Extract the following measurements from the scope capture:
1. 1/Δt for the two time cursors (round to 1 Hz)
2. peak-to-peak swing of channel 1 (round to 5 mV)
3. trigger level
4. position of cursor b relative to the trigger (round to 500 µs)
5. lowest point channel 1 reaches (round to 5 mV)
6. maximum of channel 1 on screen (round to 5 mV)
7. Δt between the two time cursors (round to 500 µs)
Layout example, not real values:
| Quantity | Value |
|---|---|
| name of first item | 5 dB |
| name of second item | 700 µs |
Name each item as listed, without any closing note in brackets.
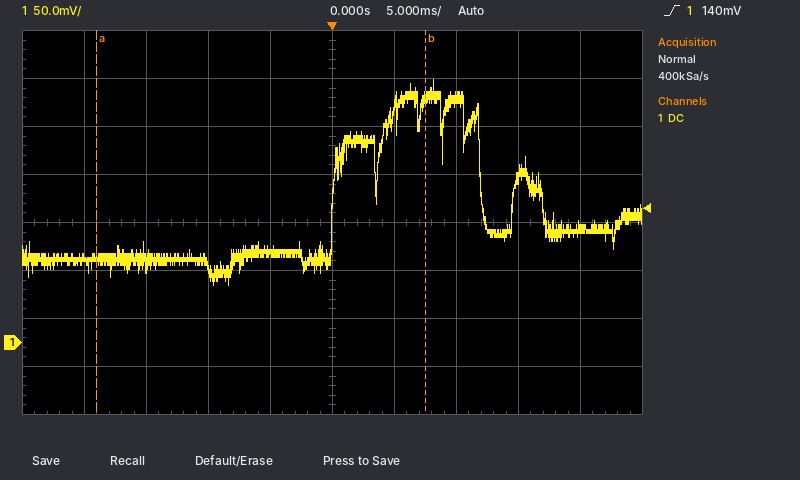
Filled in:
| Quantity | Value |
|---|---|
| 1/Δt for the two time cursors | 38 Hz |
| peak-to-peak swing of channel 1 | 215 mV |
| trigger level | 140 mV |
| position of cursor b relative to the trigger | +7.5 ms |
| lowest point channel 1 reaches | 60 mV |
| maximum of channel 1 on screen | 275 mV |
| Δt between the two time cursors | 26.5 ms |
